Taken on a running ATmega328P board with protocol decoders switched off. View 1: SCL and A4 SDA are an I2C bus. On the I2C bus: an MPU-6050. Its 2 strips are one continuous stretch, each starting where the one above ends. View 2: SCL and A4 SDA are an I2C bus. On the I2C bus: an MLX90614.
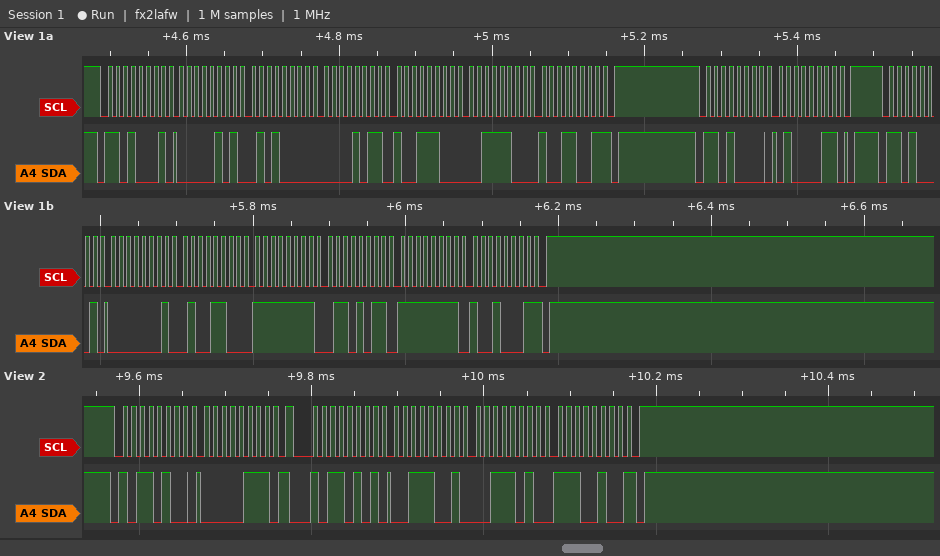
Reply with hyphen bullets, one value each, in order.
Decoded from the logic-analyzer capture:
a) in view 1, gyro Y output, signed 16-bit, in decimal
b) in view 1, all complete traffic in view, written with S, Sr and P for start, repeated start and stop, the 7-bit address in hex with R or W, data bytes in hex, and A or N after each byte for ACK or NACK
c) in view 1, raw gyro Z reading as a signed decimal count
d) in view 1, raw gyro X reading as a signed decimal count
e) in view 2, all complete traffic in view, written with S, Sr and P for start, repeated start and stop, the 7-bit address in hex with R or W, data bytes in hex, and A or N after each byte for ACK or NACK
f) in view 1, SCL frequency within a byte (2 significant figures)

- -149
- S 68R A 05 A 50 A 0B A 9C A 3C A 99 N P S 68W A 43 A P S 68R A 01 A 4C A FF A 6B A FF A 91 N P
- -111
- 332
- S 5AW A 07 A Sr 5AR A 39 A 3A A E4 N P
- 100 kHz
